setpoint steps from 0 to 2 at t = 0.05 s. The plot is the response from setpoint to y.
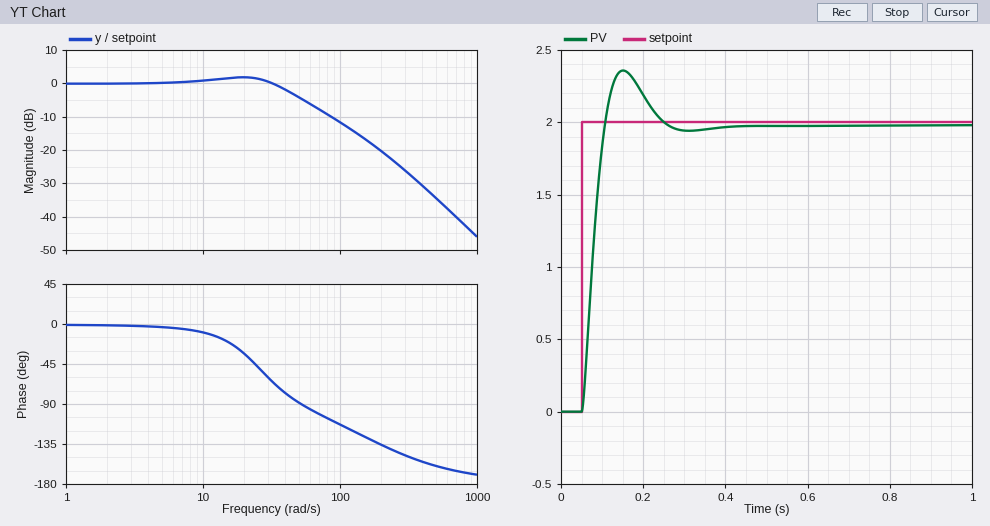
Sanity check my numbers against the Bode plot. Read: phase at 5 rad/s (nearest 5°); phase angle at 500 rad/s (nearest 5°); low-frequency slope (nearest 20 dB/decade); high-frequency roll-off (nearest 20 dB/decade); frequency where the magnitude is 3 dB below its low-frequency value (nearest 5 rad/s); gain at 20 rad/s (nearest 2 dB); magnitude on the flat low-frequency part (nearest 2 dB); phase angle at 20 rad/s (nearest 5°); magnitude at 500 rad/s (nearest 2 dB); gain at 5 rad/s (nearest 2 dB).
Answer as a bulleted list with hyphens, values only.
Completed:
- -5°
- -160°
- 0 dB/decade
- -40 dB/decade
- 45 rad/s
- 2 dB
- 0 dB
- -35°
- -34 dB
- 0 dB
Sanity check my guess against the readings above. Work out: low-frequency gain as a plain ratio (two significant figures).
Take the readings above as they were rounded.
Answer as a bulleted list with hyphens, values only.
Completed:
- 1.0
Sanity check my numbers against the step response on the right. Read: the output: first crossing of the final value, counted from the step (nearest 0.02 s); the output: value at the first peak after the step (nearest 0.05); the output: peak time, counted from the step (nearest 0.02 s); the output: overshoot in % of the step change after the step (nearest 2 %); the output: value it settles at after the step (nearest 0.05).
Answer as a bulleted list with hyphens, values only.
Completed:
- 0.06 s
- 2.35
- 0.10 s
- 18 %
- 2.00
